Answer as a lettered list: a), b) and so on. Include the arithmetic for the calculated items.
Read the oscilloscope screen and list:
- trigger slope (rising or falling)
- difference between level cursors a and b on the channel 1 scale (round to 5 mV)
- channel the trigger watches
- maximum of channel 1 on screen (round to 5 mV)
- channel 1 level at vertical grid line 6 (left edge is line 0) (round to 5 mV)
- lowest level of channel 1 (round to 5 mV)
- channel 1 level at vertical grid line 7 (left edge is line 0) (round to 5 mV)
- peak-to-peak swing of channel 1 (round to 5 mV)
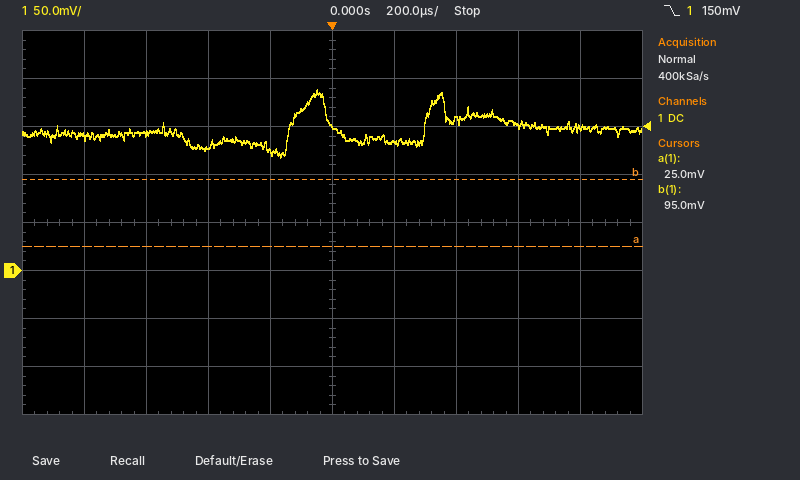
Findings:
a) falling
b) 70 mV
c) channel 1
d) 190 mV
e) 135 mV
f) 120 mV
g) 155 mV
h) 190 mV − (120 mV) = 70 mV
